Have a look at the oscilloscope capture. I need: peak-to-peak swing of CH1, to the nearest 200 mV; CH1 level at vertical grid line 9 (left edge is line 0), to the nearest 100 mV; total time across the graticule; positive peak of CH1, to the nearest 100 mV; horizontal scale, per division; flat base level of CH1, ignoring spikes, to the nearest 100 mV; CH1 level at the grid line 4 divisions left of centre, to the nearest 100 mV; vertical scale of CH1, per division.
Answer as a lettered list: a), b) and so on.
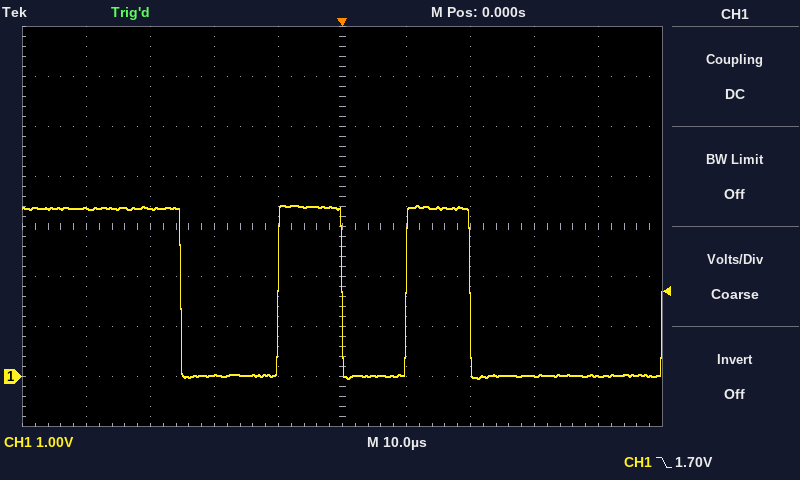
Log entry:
a) 3.4 V
b) 0.0 V
c) 100 µs
d) 3.4 V
e) 10 µs
f) 0.0 V
g) 3.4 V
h) 1 V
